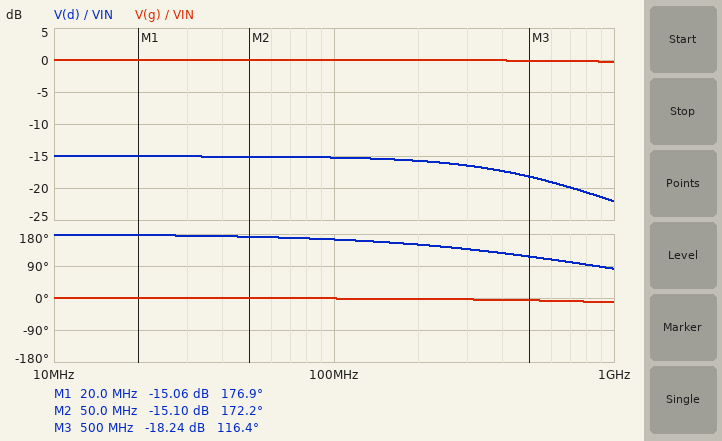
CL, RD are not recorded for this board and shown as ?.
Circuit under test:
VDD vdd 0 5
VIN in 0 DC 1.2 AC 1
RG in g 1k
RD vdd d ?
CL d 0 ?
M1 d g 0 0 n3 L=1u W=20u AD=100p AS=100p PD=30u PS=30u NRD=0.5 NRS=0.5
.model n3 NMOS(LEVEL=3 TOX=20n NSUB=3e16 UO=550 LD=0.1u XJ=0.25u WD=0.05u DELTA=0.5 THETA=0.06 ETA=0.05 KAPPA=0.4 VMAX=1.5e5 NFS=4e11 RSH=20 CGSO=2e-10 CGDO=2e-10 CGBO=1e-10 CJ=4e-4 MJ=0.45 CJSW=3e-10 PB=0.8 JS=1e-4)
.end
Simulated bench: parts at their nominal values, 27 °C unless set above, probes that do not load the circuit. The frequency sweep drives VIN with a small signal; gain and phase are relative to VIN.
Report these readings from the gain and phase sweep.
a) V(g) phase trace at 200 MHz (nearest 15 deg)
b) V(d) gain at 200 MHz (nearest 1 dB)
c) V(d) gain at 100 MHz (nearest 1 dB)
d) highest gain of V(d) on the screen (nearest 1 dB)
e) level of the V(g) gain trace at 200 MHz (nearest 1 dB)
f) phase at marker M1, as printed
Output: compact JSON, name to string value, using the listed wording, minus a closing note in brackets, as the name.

{"V(g) phase trace at 200 MHz": "0 deg", "V(d) gain at 200 MHz": "-16 dB", "V(d) gain at 100 MHz": "-15 dB", "highest gain of V(d) on the screen": "-15 dB", "level of the V(g) gain trace at 200 MHz": "0 dB", "phase at marker M1, as printed": "176.9 deg"}
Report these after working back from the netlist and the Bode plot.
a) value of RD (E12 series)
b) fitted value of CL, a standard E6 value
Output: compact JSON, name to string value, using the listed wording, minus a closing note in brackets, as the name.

{"value of RD": "18 kΩ", "fitted value of CL, a standard E6 value": "470 fF"}
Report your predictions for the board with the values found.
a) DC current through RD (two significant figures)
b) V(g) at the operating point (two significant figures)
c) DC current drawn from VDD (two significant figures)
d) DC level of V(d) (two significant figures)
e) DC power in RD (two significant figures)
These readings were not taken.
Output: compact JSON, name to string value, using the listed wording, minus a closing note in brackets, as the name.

{"DC current through RD": "270 µA", "V(g) at the operating point": "1.2 V", "DC current drawn from VDD": "270 µA", "DC level of V(d)": "150 mV", "DC power in RD": "1.3 mW"}
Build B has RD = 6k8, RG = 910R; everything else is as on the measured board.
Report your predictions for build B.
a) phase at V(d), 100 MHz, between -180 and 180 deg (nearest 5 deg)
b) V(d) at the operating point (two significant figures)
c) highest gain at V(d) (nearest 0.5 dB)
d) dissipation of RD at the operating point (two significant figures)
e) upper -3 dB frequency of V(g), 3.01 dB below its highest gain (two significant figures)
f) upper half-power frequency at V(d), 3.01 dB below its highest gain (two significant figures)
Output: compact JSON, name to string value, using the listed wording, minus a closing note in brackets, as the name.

{"phase at V(d), 100 MHz, between -180 and 180 deg": "150 deg", "V(d) at the operating point": "550 mV", "highest gain at V(d)": "3.5 dB", "dissipation of RD at the operating point": "2.9 mW", "upper -3 dB frequency of V(g), 3.01 dB below its highest gain": "5.4 GHz", "upper half-power frequency at V(d), 3.01 dB below its highest gain": "190 MHz"}
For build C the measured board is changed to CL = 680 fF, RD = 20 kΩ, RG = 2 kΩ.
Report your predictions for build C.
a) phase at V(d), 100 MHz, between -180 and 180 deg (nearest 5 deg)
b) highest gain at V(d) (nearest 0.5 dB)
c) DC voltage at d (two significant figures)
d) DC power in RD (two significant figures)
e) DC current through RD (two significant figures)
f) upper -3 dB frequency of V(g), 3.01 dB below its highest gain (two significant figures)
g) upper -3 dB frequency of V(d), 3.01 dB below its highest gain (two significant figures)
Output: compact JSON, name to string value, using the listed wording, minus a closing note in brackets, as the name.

{"phase at V(d), 100 MHz, between -180 and 180 deg": "160 deg", "highest gain at V(d)": "-16.5 dB", "DC voltage at d": "130 mV", "DC power in RD": "1.2 mW", "DC current through RD": "240 µA", "upper -3 dB frequency of V(g), 3.01 dB below its highest gain": "2.2 GHz", "upper -3 dB frequency of V(d), 3.01 dB below its highest gain": "350 MHz"}
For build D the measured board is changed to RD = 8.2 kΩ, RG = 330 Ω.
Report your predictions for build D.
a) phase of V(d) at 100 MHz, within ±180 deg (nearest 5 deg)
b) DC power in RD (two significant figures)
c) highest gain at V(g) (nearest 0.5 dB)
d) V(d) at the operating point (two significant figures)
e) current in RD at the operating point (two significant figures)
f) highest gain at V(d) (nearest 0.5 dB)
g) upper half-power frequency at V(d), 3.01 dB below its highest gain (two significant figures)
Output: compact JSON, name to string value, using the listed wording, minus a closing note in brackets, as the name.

{"phase of V(d) at 100 MHz, within ±180 deg": "160 deg", "DC power in RD": "2.6 mW", "highest gain at V(g)": "0 dB", "V(d) at the operating point": "400 mV", "current in RD at the operating point": "560 µA", "highest gain at V(d)": "-2.5 dB", "upper half-power frequency at V(d), 3.01 dB below its highest gain": "280 MHz"}
